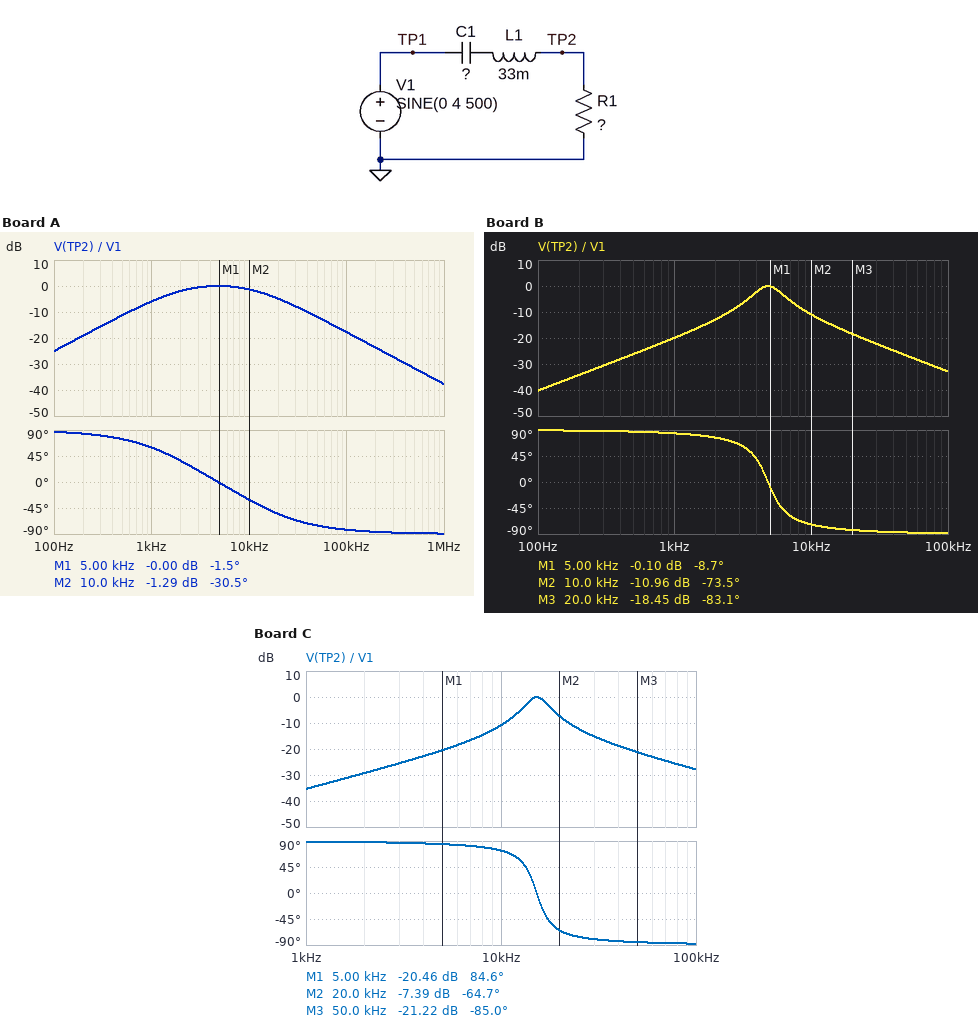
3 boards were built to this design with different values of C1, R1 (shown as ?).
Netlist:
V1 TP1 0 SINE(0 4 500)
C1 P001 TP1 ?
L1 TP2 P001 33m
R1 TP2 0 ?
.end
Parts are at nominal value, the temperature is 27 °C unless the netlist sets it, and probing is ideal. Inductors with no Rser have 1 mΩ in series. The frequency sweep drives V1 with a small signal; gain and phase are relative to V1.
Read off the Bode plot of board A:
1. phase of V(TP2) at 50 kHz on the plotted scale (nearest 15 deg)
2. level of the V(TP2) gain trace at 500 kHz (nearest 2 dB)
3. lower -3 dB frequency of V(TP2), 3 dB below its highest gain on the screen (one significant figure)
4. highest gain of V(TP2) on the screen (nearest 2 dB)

-75 deg
-32 dB
2 kHz
0 dB
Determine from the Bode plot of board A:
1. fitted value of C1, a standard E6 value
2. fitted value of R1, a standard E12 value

33 nF
2.7 kΩ
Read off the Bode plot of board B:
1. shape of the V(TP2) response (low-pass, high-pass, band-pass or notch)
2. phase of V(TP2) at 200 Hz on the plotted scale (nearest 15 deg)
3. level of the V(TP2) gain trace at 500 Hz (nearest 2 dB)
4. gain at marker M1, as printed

band-pass
90 deg
-26 dB
-0.10 dB
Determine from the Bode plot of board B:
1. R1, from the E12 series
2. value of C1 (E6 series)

470 Ω
33 nF
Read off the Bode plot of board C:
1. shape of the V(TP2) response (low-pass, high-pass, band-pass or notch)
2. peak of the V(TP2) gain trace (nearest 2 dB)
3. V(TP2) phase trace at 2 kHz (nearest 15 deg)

band-pass
0 dB
90 deg
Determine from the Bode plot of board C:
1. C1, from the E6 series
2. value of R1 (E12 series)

3.3 nF
820 Ω
